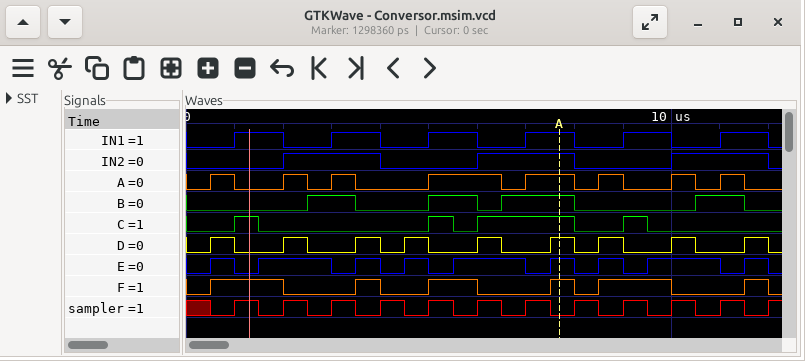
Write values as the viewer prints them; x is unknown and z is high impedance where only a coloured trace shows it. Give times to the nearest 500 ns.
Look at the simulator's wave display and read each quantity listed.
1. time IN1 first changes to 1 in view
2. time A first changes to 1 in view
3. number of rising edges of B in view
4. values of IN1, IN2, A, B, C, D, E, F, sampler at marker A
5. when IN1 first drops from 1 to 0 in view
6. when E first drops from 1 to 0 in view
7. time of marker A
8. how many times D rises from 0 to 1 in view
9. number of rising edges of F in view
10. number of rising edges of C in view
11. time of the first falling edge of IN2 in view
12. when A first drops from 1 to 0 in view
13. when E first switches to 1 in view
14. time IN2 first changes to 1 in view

1000 ns
500 ns
4
IN1=1, IN2=1, A=1, B=1, C=1, D=1, E=1, F=1, sampler=0
2000 ns
1000 ns
7500 ns
9
6
4
4000 ns
1000 ns
500 ns
2000 ns
